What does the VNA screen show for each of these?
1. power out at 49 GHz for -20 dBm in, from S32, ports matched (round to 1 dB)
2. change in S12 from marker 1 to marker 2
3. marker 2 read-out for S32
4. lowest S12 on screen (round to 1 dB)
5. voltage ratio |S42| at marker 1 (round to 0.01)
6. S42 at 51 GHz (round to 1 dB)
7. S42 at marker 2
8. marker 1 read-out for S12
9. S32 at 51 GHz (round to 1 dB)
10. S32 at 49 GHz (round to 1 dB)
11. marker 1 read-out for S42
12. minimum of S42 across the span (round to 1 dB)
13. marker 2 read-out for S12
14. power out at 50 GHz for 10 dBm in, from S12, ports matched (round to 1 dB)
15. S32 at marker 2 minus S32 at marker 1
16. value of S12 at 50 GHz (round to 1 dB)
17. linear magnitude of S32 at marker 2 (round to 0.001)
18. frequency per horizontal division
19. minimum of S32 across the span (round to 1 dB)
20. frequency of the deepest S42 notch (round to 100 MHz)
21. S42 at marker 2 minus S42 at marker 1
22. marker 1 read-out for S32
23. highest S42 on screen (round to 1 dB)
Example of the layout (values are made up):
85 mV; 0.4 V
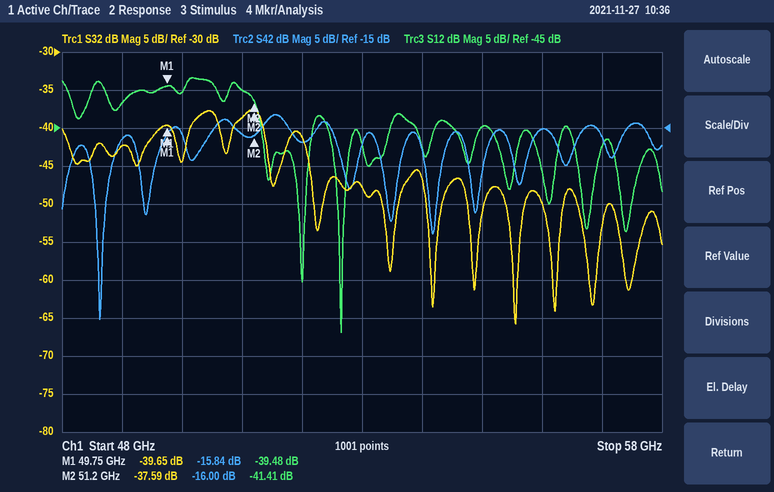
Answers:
-62 dBm; -1.93 dB; -37.59 dB; -72 dB; 0.16; -16 dB; -16.00 dB; -39.48 dB; -39 dB; -42 dB; -15.84 dB; -40 dB; -41.41 dB; -30 dBm; 2.06 dB; -40 dB; 0.013; 1 GHz; -66 dB; 48.6 GHz; -0.16 dB; -39.65 dB; -13 dB
